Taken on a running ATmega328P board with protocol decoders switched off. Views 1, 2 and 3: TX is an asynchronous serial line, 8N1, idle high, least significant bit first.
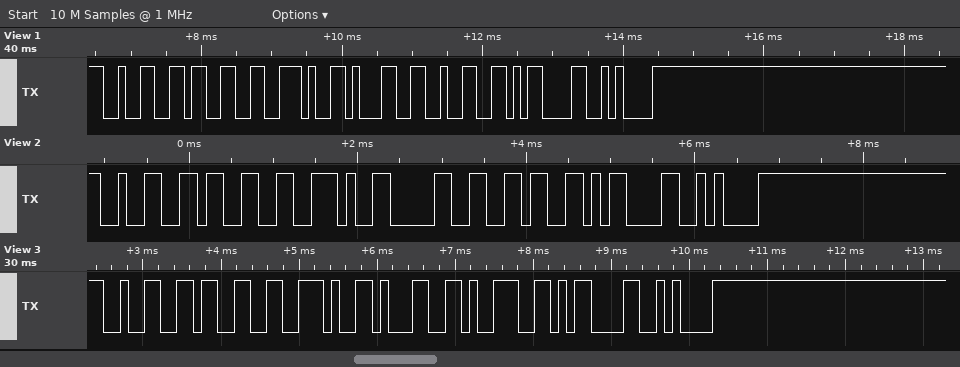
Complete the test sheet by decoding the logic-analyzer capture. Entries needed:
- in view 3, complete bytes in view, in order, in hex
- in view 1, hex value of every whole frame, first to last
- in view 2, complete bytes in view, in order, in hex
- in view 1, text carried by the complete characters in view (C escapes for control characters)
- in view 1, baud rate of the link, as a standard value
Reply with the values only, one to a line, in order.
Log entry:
32 33 2E 31 39 0D 0A
32 33 2E 31 32 0D 0A
32 33 2E 30 36 0D 0A
"23.12\r\n"
9600 baud
